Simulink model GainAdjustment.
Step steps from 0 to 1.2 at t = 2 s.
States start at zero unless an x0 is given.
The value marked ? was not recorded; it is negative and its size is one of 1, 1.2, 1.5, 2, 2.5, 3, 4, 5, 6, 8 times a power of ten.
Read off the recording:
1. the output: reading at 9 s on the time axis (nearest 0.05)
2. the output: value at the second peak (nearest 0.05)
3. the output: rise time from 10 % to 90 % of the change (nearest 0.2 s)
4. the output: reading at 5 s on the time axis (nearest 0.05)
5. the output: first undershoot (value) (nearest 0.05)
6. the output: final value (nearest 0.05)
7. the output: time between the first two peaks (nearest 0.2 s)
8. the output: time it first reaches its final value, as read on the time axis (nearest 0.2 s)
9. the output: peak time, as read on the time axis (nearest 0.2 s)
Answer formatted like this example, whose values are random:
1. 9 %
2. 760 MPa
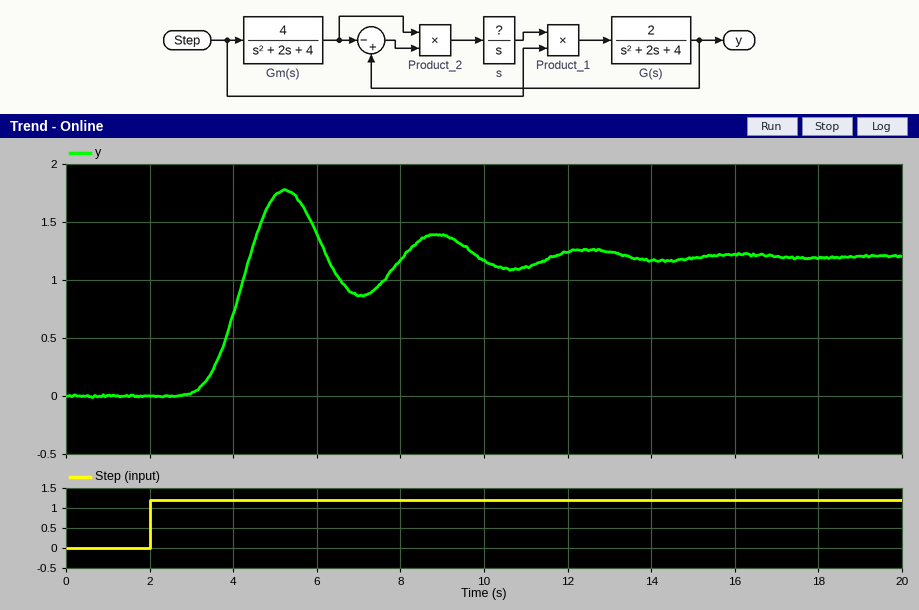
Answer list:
1. 1.40
2. 1.40
3. 1.0 s
4. 1.75
5. 0.85
6. 1.20
7. 3.6 s
8. 4.4 s
9. 5.2 s
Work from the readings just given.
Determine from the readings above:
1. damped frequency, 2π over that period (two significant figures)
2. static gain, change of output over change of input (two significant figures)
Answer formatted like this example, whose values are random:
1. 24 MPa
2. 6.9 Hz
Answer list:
1. 1.7 rad/s
2. 1.0
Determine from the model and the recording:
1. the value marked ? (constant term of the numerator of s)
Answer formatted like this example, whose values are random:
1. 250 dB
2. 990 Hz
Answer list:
1. -1.5
